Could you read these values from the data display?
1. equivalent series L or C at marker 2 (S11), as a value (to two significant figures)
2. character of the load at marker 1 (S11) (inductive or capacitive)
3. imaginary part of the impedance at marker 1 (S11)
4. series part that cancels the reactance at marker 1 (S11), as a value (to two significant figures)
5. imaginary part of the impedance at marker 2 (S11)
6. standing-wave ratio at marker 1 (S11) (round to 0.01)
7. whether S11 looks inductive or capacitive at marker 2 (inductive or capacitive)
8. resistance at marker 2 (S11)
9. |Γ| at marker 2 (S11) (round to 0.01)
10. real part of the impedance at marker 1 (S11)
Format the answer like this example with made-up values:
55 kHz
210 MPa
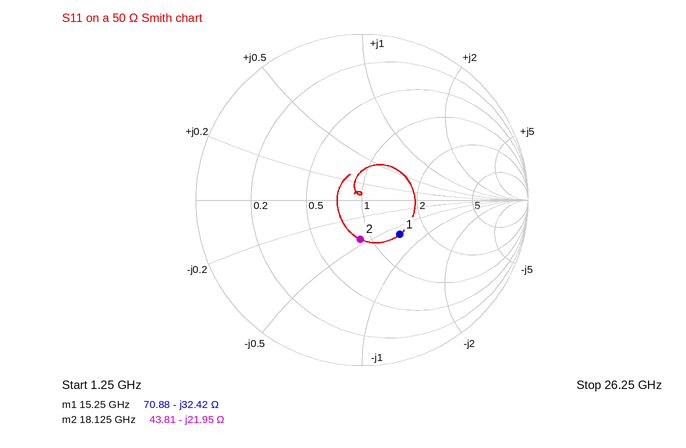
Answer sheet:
400 fF
capacitive
-32.42 Ω
340 pH
-21.95 Ω
1.89
capacitive
43.81 Ω
0.24
70.88 Ω
